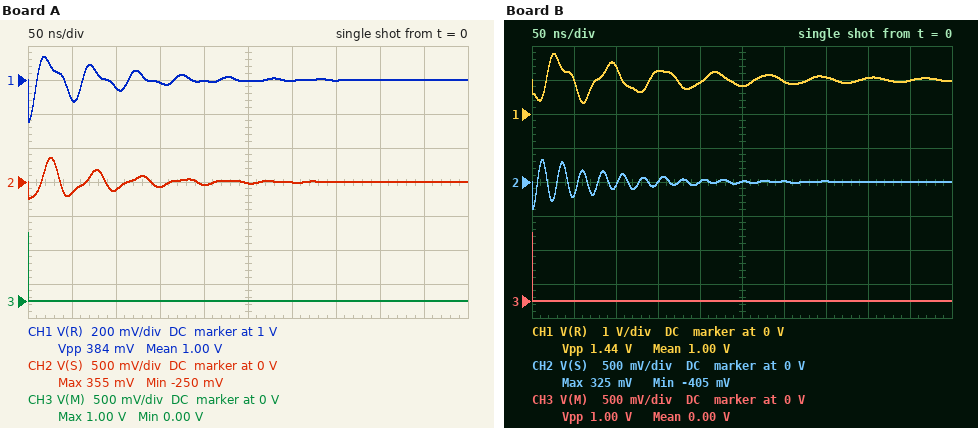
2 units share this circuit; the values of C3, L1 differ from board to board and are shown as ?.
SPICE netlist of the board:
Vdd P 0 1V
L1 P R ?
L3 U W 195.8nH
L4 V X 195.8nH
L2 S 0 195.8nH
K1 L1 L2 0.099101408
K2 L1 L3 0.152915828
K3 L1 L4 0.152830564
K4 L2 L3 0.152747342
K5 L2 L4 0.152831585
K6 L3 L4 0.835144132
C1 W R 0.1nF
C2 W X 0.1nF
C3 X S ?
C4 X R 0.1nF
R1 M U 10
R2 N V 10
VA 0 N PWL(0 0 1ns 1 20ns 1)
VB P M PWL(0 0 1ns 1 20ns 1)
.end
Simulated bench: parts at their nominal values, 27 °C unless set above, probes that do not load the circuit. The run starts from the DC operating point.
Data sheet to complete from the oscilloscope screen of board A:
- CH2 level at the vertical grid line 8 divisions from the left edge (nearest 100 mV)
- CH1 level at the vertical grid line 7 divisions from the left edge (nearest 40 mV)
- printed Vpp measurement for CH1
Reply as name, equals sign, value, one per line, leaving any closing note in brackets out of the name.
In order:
CH2 level at the vertical grid line 8 divisions from the left edge = 0 V
CH1 level at the vertical grid line 7 divisions from the left edge = 1.00 V
printed Vpp measurement for CH1 = 384 mV
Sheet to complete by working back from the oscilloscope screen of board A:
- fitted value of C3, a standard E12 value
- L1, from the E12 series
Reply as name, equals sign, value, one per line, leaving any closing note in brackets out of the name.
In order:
fitted value of C3, a standard E12 value = 82 pF
L1, from the E12 series = 100 nH
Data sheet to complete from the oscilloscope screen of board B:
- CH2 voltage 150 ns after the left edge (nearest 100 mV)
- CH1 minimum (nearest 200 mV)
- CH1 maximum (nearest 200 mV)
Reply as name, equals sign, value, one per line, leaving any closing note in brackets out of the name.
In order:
CH2 voltage 150 ns after the left edge = 0 V
CH1 minimum = 400 mV
CH1 maximum = 1.8 V
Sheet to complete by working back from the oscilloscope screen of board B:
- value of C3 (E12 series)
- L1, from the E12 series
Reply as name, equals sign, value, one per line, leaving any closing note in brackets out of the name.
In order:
value of C3 = 39 pF
L1, from the E12 series = 390 nH
